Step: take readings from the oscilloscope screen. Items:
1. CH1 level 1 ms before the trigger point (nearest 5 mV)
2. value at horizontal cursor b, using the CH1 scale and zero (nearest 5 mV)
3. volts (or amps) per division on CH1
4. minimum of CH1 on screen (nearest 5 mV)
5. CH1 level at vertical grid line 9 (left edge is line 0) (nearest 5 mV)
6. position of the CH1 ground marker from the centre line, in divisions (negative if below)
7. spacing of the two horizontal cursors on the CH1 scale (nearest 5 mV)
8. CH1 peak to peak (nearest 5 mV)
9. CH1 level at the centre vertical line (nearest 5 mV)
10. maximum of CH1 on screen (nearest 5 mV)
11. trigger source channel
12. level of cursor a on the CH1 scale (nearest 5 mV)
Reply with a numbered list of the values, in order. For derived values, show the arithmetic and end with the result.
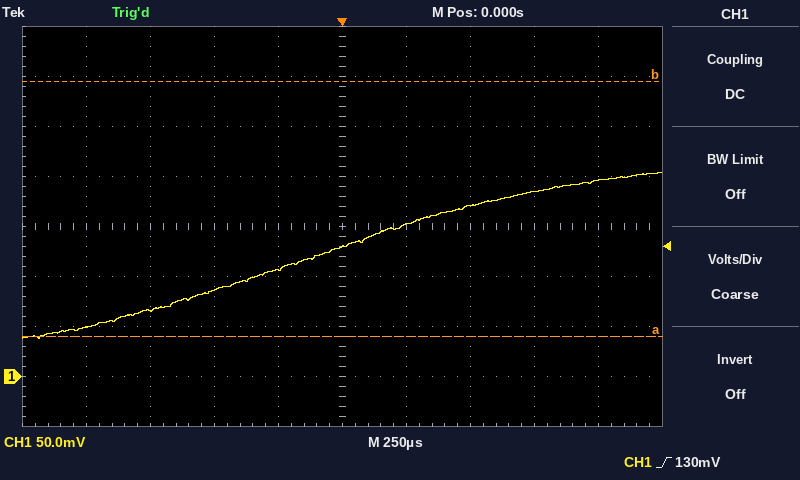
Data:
1. 50 mV
2. 295 mV
3. 50 mV
4. 40 mV
5. 195 mV
6. -3.0 div
7. 255 mV
8. 205 mV − (40 mV) = 165 mV
9. 130 mV
10. 205 mV
11. CH1
12. 40 mV
